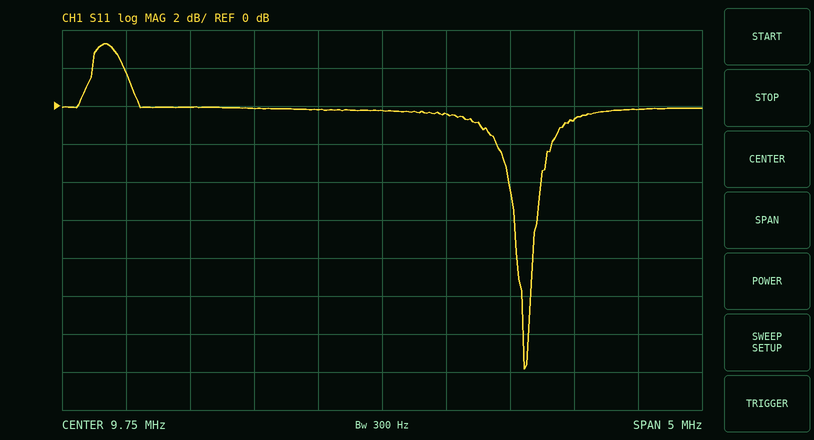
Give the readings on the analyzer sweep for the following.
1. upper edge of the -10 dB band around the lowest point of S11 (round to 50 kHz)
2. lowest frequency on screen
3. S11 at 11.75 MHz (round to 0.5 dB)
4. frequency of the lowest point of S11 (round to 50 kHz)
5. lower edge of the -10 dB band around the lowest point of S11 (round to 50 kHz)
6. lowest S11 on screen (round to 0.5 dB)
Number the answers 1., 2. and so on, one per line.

1. 10.90 MHz
2. 7.25 MHz
3. 0.0 dB
4. 10.85 MHz
5. 10.85 MHz
6. -14.0 dB
